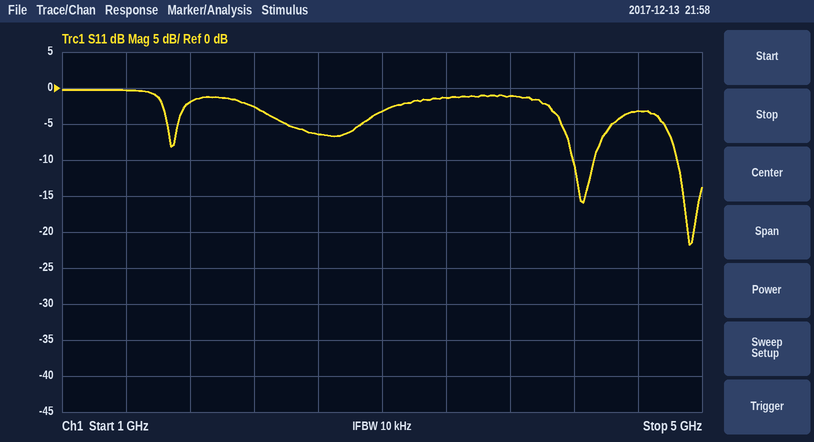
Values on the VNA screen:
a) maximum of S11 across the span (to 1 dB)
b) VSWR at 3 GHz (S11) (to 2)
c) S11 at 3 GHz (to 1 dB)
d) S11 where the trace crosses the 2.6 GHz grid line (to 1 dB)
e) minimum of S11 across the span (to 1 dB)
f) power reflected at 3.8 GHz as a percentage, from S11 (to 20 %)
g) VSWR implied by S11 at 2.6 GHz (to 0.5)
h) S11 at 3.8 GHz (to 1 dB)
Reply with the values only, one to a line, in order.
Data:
0 dB
6
-3 dB
-6 dB
-22 dB
80 %
3.0
-1 dB
